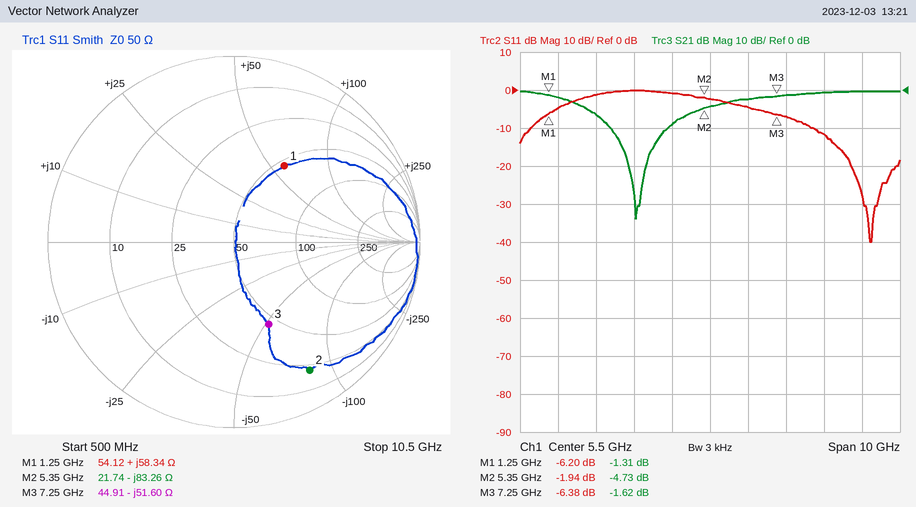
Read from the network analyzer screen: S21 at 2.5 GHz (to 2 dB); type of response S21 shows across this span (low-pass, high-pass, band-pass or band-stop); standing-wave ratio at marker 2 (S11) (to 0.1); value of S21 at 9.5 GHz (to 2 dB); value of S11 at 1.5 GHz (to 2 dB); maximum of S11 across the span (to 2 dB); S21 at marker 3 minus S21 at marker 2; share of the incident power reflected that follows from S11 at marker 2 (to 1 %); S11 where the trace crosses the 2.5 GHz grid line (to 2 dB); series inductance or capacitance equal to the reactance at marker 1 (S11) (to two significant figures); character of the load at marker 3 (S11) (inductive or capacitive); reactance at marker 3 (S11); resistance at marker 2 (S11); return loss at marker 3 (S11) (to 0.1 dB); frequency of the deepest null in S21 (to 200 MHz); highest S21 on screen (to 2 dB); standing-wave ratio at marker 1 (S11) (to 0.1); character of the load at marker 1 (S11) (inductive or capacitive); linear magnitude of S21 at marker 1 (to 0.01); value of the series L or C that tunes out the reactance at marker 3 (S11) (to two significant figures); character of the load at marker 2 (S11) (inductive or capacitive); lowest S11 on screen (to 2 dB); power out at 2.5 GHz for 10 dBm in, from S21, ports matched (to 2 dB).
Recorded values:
-6 dB
band-stop
9.0
0 dB
-4 dB
0 dB
3.11 dB
64 %
-2 dB
7.4 nH
capacitive
-51.60 Ω
21.74 Ω
6.4 dB
3.6 GHz
0 dB
2.9
inductive
0.86
1.1 nH
capacitive
-40 dB
4 dBm
